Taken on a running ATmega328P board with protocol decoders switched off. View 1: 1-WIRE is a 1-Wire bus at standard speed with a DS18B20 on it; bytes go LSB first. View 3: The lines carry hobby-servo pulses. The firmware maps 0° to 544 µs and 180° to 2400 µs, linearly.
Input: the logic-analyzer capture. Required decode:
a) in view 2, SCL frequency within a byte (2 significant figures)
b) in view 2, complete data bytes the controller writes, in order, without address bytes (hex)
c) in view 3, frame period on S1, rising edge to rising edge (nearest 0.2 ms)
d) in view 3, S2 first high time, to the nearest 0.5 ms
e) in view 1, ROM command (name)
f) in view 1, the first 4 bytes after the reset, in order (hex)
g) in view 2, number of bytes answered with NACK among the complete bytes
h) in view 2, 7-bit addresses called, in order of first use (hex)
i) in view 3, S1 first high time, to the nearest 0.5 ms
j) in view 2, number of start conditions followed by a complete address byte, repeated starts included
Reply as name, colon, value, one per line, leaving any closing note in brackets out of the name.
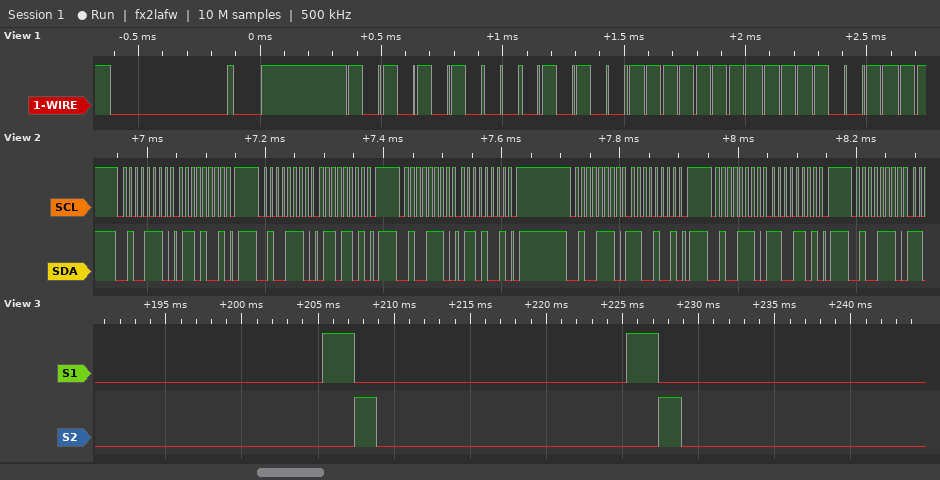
in view 2, SCL frequency within a byte: 100 kHz
in view 2, complete data bytes the controller writes, in order, without address bytes: 69 6D 69 C9 CD
in view 3, frame period on S1, rising edge to rising edge: 20.0 ms
in view 3, S2 first high time, to the nearest 0.5 ms: 1.5 ms
in view 1, ROM command: Match ROM
in view 1, the first 4 bytes after the reset, in order: 55 28 FF CF
in view 2, number of bytes answered with NACK among the complete bytes: 0
in view 2, 7-bit addresses called, in order of first use: 0x27
in view 3, S1 first high time, to the nearest 0.5 ms: 2.0 ms
in view 2, number of start conditions followed by a complete address byte, repeated starts included: 6
